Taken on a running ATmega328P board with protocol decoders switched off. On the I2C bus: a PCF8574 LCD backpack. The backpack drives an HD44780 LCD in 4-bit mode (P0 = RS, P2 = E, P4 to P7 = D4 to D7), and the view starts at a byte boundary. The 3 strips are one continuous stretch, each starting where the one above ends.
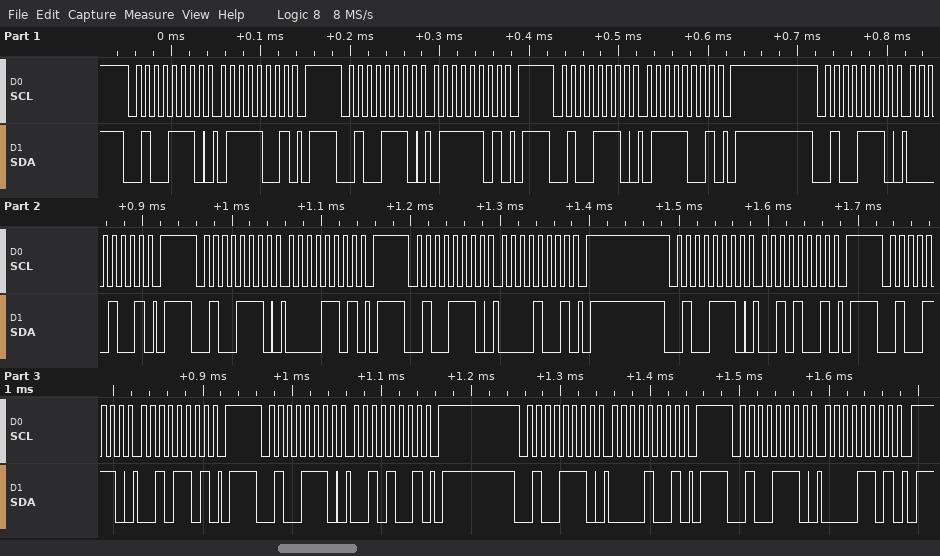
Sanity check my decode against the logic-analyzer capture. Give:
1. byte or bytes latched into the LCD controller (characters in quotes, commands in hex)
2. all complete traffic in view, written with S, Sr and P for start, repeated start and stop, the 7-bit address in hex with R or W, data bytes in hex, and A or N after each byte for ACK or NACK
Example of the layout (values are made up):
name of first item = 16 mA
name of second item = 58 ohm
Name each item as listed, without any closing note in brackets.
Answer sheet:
byte or bytes latched into the LCD controller = 'p'
all complete traffic in view, written with S, Sr and P for start, repeated start and stop, the 7-bit address in hex with R or W, data bytes in hex, and A or N after each byte for ACK or NACK = S 27W A 79 A P S 27W A 7D A P S 27W A 79 A P S 27W A 09 A P S 27W A 0D A P S 27W A 09 A P S 27W A 29 A P S 27W A 2D A P S 27W A 29 A P S 27W A 09 A P S 27W A 0D A P
